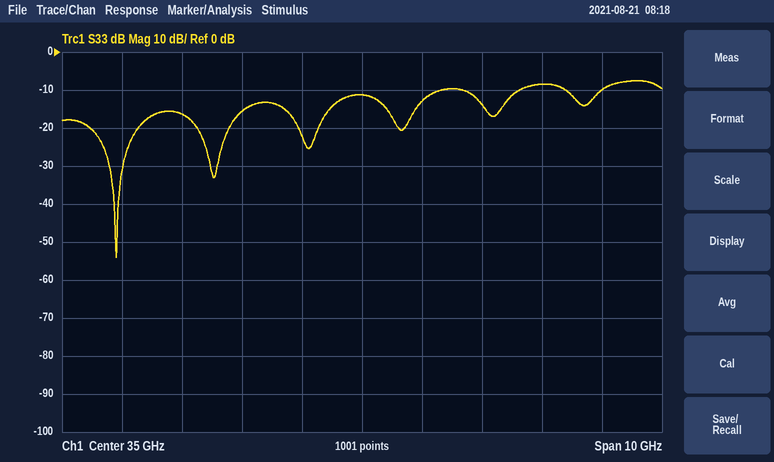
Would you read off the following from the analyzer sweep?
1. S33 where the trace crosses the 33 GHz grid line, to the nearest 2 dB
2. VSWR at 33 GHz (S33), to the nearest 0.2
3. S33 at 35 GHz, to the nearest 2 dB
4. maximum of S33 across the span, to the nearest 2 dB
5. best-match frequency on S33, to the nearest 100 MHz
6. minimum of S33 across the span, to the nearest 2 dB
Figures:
-16 dB
1.4
-12 dB
-8 dB
30.9 GHz
-54 dB
